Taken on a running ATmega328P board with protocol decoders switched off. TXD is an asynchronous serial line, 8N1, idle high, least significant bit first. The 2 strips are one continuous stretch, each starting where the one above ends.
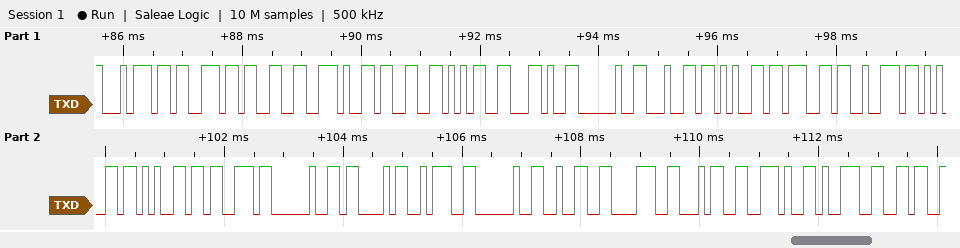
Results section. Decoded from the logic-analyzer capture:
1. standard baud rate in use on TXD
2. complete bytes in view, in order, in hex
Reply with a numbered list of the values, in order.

1. 9600 baud
2. 0x74 0x73 0x33 0x2E 0x33 0x35 0x2C 0x20 0x64 0x65 0x67 0x72 0x65 0x65 0x73 0x20 0x43 0x3A 0x20 0x32 0x38 0x34 0x2E 0x39 0x36
